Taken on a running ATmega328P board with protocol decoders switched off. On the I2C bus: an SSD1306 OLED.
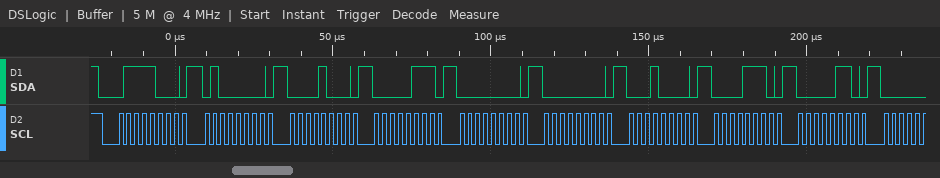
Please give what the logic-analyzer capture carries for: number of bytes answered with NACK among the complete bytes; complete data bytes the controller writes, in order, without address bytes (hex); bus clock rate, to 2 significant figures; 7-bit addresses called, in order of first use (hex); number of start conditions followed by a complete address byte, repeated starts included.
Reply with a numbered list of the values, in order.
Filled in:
1. 0
2. 40 08 07 00 00 10 0E 06
3. 400 kHz
4. 0x3C
5. 1
